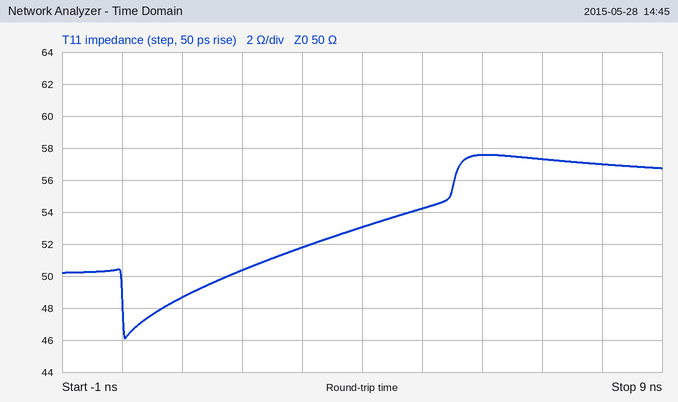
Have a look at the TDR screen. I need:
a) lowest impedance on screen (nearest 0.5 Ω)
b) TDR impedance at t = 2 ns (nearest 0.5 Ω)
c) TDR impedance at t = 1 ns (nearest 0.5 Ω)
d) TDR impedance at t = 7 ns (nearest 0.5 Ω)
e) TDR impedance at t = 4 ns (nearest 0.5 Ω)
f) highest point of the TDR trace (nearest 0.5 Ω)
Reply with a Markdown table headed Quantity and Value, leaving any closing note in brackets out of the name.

| Quantity | Value |
|---|---|
| lowest impedance on screen | 46.0 Ω |
| TDR impedance at t = 2 ns | 50.5 Ω |
| TDR impedance at t = 1 ns | 48.5 Ω |
| TDR impedance at t = 7 ns | 57.5 Ω |
| TDR impedance at t = 4 ns | 53.0 Ω |
| highest point of the TDR trace | 57.5 Ω |
